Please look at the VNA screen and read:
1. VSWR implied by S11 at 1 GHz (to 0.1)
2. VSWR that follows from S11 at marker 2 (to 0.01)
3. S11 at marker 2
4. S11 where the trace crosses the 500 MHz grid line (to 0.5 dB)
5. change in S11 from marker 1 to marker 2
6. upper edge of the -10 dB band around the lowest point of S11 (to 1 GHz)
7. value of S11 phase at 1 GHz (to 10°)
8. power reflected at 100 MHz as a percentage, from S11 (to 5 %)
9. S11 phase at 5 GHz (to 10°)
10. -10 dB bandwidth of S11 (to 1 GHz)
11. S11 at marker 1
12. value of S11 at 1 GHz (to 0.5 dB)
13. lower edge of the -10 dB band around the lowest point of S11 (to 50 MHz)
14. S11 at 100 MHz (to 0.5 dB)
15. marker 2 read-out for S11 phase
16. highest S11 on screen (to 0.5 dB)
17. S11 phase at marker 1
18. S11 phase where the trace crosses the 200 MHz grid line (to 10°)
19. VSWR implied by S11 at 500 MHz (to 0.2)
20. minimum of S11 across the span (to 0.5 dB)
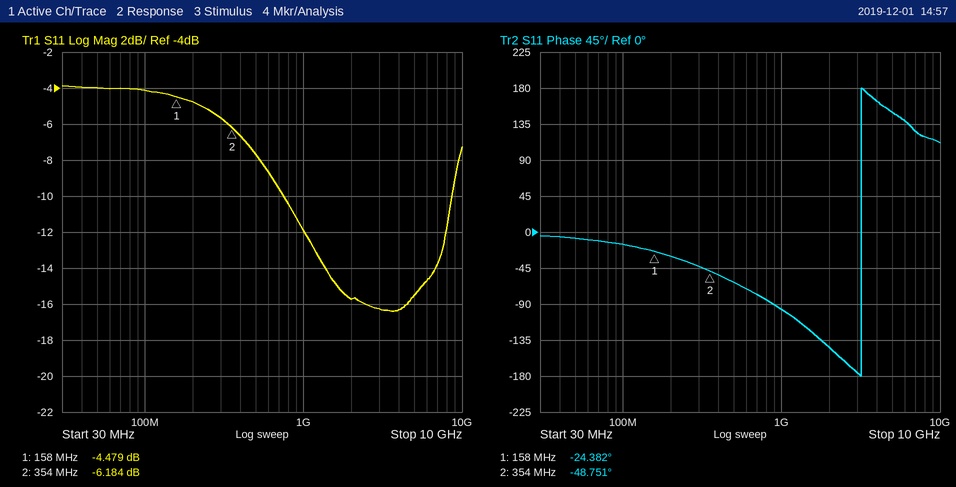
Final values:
1.7
2.93
-6.184 dB
-7.5 dB
-1.705 dB
9 GHz
-100°
40 %
150°
8 GHz
-4.479 dB
-12.0 dB
750 MHz
-4.0 dB
-48.751°
-4.0 dB
-24.382°
-30°
2.4
-16.5 dB
